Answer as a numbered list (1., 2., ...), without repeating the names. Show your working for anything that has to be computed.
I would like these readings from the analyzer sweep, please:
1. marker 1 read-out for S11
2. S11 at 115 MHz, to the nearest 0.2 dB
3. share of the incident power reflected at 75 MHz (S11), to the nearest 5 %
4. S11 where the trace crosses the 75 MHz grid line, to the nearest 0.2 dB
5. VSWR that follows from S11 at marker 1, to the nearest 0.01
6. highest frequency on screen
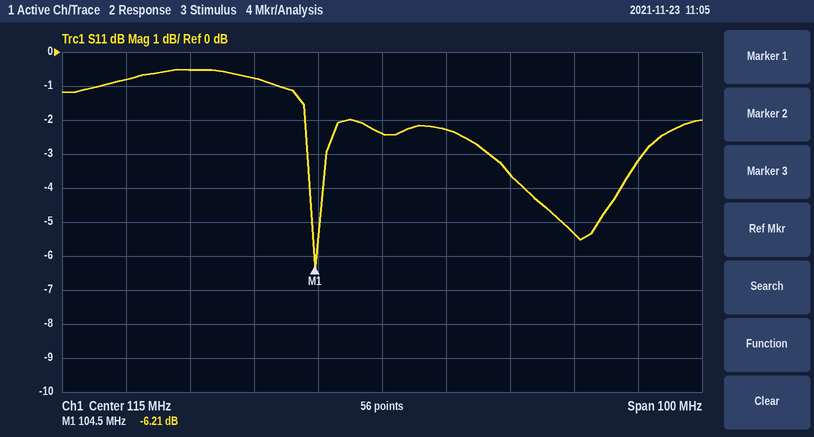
1. -6.21 dB
2. -2.4 dB
3. 10^(-0.8/10) ≈ 83.2 %, so 85 % to the nearest 5 %
4. -0.8 dB
5. (1 + 0.4892)/(1 − 0.4892) ≈ 2.92
6. 165 MHz
